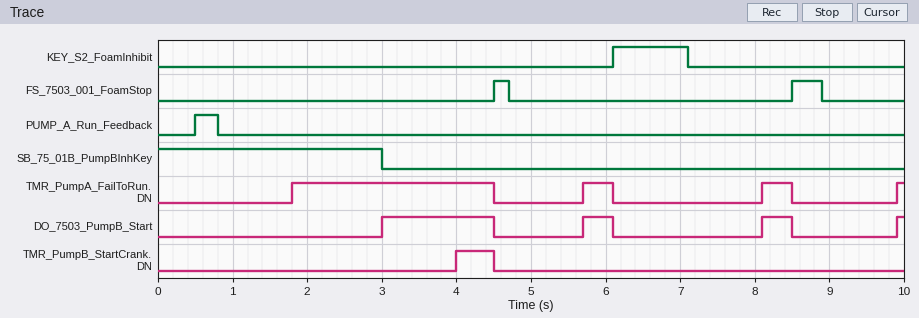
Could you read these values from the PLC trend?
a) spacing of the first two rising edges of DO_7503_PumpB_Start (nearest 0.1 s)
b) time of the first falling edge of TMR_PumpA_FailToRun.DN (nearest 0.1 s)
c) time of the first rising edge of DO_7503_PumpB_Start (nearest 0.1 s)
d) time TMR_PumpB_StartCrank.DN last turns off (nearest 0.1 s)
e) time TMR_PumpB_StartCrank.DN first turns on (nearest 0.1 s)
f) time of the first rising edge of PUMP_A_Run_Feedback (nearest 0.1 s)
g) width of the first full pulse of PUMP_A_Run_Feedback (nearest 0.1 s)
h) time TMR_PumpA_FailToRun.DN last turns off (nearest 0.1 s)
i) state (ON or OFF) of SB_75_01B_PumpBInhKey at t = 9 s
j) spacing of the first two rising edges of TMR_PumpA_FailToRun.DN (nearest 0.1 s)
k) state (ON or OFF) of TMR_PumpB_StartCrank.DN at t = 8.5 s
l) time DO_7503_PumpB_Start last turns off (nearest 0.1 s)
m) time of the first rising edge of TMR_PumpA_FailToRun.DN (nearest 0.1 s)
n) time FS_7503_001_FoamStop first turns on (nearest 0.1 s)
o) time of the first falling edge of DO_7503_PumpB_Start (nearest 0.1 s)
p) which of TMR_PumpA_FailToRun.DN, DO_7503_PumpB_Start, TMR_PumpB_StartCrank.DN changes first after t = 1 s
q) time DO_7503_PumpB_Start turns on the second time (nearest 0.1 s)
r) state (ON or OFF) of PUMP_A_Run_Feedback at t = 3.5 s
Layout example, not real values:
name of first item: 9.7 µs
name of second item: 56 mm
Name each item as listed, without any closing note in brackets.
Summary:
spacing of the first two rising edges of DO_7503_PumpB_Start: 2.7 s
time of the first falling edge of TMR_PumpA_FailToRun.DN: 4.5 s
time of the first rising edge of DO_7503_PumpB_Start: 3.0 s
time TMR_PumpB_StartCrank.DN last turns off: 4.5 s
time TMR_PumpB_StartCrank.DN first turns on: 4.0 s
time of the first rising edge of PUMP_A_Run_Feedback: 0.5 s
width of the first full pulse of PUMP_A_Run_Feedback: 0.3 s
time TMR_PumpA_FailToRun.DN last turns off: 8.5 s
state (ON or OFF) of SB_75_01B_PumpBInhKey at t = 9 s: OFF
spacing of the first two rising edges of TMR_PumpA_FailToRun.DN: 3.9 s
state (ON or OFF) of TMR_PumpB_StartCrank.DN at t = 8.5 s: OFF
time DO_7503_PumpB_Start last turns off: 8.5 s
time of the first rising edge of TMR_PumpA_FailToRun.DN: 1.8 s
time FS_7503_001_FoamStop first turns on: 4.5 s
time of the first falling edge of DO_7503_PumpB_Start: 4.5 s
which of TMR_PumpA_FailToRun.DN, DO_7503_PumpB_Start, TMR_PumpB_StartCrank.DN changes first after t = 1 s: TMR_PumpA_FailToRun.DN
time DO_7503_PumpB_Start turns on the second time: 5.7 s
state (ON or OFF) of PUMP_A_Run_Feedback at t = 3.5 s: OFF
